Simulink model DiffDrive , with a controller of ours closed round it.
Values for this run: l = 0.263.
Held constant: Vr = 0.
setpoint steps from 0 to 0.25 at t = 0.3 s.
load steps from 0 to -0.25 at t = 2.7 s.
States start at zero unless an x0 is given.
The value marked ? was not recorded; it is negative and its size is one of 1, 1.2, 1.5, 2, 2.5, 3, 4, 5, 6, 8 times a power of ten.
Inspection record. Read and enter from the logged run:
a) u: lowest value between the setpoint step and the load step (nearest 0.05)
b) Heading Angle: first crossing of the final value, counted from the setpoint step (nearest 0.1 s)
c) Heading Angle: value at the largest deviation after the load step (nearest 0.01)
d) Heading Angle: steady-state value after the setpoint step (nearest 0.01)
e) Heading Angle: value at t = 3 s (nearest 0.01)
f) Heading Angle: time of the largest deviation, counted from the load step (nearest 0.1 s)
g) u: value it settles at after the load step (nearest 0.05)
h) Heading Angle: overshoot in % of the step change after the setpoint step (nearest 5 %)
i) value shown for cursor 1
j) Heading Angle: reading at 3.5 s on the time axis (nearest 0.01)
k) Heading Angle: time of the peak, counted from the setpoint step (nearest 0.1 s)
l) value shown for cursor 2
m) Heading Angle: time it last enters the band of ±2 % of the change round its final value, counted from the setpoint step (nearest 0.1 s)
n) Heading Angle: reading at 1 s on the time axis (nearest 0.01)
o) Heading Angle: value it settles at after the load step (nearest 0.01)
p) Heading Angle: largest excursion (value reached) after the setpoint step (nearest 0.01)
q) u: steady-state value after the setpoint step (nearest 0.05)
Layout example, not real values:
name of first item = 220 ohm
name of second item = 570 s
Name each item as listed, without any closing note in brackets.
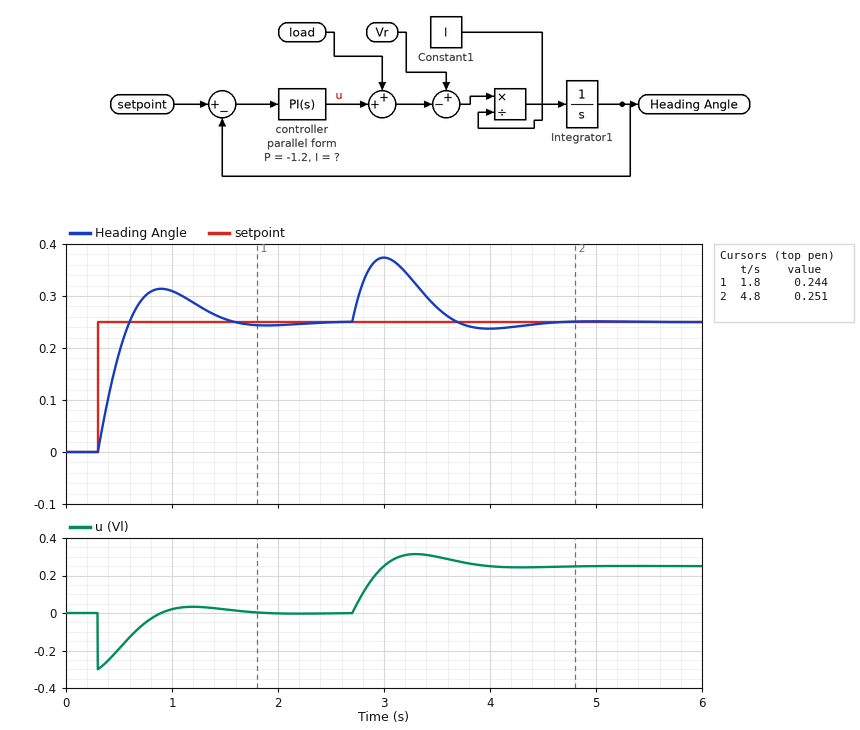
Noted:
u: lowest value between the setpoint step and the load step = -0.30
Heading Angle: first crossing of the final value, counted from the setpoint step = 0.3 s
Heading Angle: value at the largest deviation after the load step = 0.37
Heading Angle: steady-state value after the setpoint step = 0.25
Heading Angle: value at t = 3 s = 0.37
Heading Angle: time of the largest deviation, counted from the load step = 0.3 s
u: value it settles at after the load step = 0.25
Heading Angle: overshoot in % of the step change after the setpoint step = 25 %
value shown for cursor 1 = 0.244
Heading Angle: reading at 3.5 s on the time axis = 0.28
Heading Angle: time of the peak, counted from the setpoint step = 0.6 s
value shown for cursor 2 = 0.251
Heading Angle: time it last enters the band of ±2 % of the change round its final value, counted from the setpoint step = 1.8 s
Heading Angle: reading at 1 s on the time axis = 0.31
Heading Angle: value it settles at after the load step = 0.25
Heading Angle: largest excursion (value reached) after the setpoint step = 0.31
u: steady-state value after the setpoint step = 0.00
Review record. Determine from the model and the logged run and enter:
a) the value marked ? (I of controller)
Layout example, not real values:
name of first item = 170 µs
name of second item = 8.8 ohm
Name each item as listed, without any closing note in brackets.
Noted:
the value marked ? = -4
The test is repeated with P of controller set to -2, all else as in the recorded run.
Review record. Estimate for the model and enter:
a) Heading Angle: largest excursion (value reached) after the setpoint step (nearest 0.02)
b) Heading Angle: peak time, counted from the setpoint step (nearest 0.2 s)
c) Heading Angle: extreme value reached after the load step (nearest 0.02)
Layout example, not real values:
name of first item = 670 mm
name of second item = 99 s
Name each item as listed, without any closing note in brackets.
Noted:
Heading Angle: largest excursion (value reached) after the setpoint step = 0.28
Heading Angle: peak time, counted from the setpoint step = 0.6 s
Heading Angle: extreme value reached after the load step = 0.34
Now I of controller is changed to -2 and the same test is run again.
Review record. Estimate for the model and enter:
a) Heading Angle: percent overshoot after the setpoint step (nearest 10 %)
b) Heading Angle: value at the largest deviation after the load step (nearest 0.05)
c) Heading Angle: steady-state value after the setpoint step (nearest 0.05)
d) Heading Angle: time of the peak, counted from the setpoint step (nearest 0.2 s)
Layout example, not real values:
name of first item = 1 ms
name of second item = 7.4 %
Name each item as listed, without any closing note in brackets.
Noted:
Heading Angle: percent overshoot after the setpoint step = 20 %
Heading Angle: value at the largest deviation after the load step = 0.40
Heading Angle: steady-state value after the setpoint step = 0.25
Heading Angle: time of the peak, counted from the setpoint step = 0.8 s
